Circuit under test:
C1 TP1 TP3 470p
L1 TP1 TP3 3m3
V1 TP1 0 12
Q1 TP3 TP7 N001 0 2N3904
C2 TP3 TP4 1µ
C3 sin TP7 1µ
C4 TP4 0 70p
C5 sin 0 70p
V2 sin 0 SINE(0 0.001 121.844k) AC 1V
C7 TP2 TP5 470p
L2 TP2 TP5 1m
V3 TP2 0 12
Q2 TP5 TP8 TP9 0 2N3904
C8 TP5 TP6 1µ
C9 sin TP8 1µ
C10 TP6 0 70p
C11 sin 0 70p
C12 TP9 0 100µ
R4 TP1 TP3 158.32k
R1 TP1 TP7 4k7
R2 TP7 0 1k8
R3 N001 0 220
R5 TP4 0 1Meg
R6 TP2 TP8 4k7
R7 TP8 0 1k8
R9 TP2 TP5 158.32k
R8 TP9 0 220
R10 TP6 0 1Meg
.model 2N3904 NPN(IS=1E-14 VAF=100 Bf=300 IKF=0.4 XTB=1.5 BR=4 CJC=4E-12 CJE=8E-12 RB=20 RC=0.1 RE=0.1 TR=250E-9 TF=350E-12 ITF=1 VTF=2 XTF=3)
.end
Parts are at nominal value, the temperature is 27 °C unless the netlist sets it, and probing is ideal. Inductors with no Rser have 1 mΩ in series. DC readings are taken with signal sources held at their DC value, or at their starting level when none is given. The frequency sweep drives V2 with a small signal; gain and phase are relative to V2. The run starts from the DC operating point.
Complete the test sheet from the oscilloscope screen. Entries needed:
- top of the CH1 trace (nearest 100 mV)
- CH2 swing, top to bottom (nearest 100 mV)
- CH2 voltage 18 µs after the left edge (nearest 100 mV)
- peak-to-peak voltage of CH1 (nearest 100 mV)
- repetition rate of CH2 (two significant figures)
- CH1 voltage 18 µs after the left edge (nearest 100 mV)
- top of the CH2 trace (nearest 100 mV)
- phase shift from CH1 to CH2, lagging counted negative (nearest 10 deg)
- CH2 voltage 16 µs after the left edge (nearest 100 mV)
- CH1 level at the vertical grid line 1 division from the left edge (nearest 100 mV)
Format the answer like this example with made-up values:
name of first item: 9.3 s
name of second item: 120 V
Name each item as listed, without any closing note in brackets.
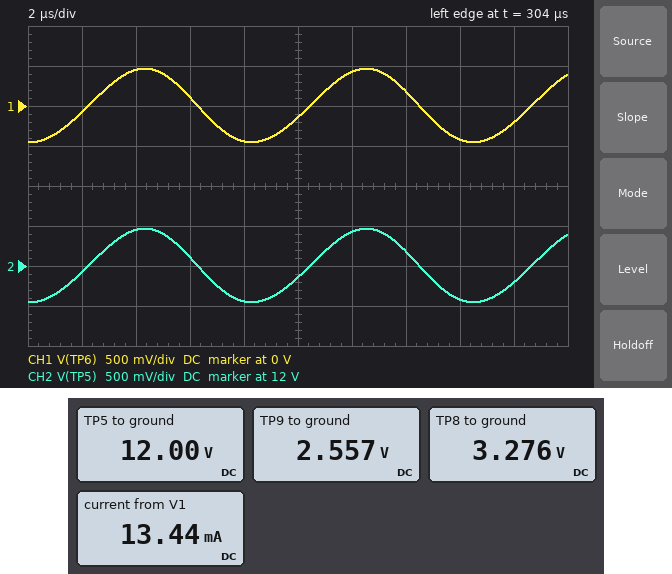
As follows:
top of the CH1 trace: 500 mV
CH2 swing, top to bottom: 900 mV
CH2 voltage 18 µs after the left edge: 11.8 V
peak-to-peak voltage of CH1: 900 mV
repetition rate of CH2: 120 kHz
CH1 voltage 18 µs after the left edge: -200 mV
top of the CH2 trace: 12.5 V
phase shift from CH1 to CH2, lagging counted negative: 0 deg
CH2 voltage 16 µs after the left edge: 11.6 V
CH1 level at the vertical grid line 1 division from the left edge: -100 mV
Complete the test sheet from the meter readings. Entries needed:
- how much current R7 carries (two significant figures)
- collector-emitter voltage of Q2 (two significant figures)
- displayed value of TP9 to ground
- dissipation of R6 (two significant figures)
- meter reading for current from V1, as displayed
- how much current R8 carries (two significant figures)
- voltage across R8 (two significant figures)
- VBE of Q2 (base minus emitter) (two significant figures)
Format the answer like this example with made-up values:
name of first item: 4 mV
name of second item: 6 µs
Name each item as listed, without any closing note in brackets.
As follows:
how much current R7 carries: 1.8 mA
collector-emitter voltage of Q2: 9.4 V
displayed value of TP9 to ground: 2.557 V
dissipation of R6: 16 mW
meter reading for current from V1, as displayed: 13.44 mA
how much current R8 carries: 12 mA
voltage across R8: 2.6 V
VBE of Q2 (base minus emitter): 720 mV
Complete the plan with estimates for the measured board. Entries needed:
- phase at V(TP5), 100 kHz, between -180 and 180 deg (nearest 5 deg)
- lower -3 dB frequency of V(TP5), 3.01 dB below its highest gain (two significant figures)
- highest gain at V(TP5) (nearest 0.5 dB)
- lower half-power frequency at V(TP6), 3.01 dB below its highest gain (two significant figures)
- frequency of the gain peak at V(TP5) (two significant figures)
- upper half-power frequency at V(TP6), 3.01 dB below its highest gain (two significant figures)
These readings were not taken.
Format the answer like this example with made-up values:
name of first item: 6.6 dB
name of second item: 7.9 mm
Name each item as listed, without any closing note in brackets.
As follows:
phase at V(TP5), 100 kHz, between -180 and 180 deg: -95 deg
lower -3 dB frequency of V(TP5), 3.01 dB below its highest gain: 200 kHz
highest gain at V(TP5): 71.5 dB
lower half-power frequency at V(TP6), 3.01 dB below its highest gain: 200 kHz
frequency of the gain peak at V(TP5): 210 kHz
upper half-power frequency at V(TP6), 3.01 dB below its highest gain: 230 kHz
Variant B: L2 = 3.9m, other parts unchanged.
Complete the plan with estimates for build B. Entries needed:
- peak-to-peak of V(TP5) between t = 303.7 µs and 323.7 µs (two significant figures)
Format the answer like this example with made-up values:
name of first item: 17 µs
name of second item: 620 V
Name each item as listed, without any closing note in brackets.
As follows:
peak-to-peak of V(TP5) between t = 303.7 µs and 323.7 µs: 5.7 V
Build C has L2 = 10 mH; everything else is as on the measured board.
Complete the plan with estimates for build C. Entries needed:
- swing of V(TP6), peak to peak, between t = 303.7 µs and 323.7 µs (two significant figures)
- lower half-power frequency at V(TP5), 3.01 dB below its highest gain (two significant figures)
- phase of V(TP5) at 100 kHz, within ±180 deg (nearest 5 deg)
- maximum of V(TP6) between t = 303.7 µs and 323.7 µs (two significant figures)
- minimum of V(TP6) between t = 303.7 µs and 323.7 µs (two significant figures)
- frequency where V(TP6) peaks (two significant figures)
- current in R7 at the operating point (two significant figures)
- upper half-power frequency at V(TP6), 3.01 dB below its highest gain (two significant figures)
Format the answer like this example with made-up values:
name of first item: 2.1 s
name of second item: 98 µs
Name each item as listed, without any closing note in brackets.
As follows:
swing of V(TP6), peak to peak, between t = 303.7 µs and 323.7 µs: 2.6 V
lower half-power frequency at V(TP5), 3.01 dB below its highest gain: 53 kHz
phase of V(TP5) at 100 kHz, within ±180 deg: 120 deg
maximum of V(TP6) between t = 303.7 µs and 323.7 µs: 1.3 V
minimum of V(TP6) between t = 303.7 µs and 323.7 µs: -1.3 V
frequency where V(TP6) peaks: 67 kHz
current in R7 at the operating point: 1.8 mA
upper half-power frequency at V(TP6), 3.01 dB below its highest gain: 85 kHz
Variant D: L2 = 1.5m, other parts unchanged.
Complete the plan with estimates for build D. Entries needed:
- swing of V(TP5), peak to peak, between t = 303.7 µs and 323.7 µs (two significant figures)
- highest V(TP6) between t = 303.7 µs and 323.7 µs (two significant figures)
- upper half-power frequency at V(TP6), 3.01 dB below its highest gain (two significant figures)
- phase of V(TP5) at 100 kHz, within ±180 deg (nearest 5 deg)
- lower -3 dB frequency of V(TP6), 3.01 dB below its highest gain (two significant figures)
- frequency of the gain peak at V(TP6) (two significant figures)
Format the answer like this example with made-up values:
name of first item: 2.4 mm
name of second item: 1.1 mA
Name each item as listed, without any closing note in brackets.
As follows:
swing of V(TP5), peak to peak, between t = 303.7 µs and 323.7 µs: 1.8 V
highest V(TP6) between t = 303.7 µs and 323.7 µs: 890 mV
upper half-power frequency at V(TP6), 3.01 dB below its highest gain: 190 kHz
phase of V(TP5) at 100 kHz, within ±180 deg: -100 deg
lower -3 dB frequency of V(TP6), 3.01 dB below its highest gain: 160 kHz
frequency of the gain peak at V(TP6): 170 kHz
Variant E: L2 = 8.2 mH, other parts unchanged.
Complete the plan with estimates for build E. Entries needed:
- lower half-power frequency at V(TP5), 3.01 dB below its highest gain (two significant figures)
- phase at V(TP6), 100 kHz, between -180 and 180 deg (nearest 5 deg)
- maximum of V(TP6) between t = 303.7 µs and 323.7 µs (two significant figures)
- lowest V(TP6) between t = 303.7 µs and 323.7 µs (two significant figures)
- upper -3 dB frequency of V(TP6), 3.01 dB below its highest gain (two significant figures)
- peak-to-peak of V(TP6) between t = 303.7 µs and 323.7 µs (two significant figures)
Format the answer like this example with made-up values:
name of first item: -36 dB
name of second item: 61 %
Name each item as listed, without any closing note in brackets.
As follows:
lower half-power frequency at V(TP5), 3.01 dB below its highest gain: 60 kHz
phase at V(TP6), 100 kHz, between -180 and 180 deg: 125 deg
maximum of V(TP6) between t = 303.7 µs and 323.7 µs: 1.4 V
lowest V(TP6) between t = 303.7 µs and 323.7 µs: -1.4 V
upper -3 dB frequency of V(TP6), 3.01 dB below its highest gain: 92 kHz
peak-to-peak of V(TP6) between t = 303.7 µs and 323.7 µs: 2.8 V
